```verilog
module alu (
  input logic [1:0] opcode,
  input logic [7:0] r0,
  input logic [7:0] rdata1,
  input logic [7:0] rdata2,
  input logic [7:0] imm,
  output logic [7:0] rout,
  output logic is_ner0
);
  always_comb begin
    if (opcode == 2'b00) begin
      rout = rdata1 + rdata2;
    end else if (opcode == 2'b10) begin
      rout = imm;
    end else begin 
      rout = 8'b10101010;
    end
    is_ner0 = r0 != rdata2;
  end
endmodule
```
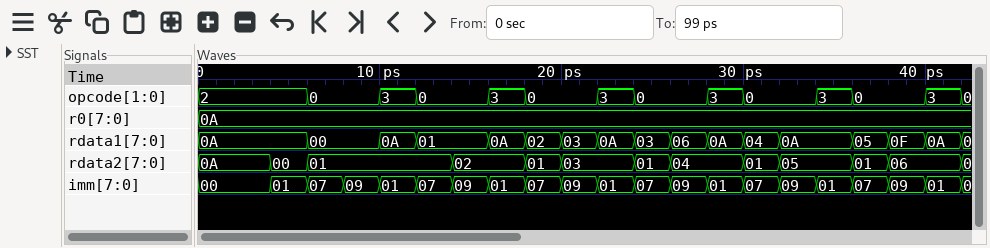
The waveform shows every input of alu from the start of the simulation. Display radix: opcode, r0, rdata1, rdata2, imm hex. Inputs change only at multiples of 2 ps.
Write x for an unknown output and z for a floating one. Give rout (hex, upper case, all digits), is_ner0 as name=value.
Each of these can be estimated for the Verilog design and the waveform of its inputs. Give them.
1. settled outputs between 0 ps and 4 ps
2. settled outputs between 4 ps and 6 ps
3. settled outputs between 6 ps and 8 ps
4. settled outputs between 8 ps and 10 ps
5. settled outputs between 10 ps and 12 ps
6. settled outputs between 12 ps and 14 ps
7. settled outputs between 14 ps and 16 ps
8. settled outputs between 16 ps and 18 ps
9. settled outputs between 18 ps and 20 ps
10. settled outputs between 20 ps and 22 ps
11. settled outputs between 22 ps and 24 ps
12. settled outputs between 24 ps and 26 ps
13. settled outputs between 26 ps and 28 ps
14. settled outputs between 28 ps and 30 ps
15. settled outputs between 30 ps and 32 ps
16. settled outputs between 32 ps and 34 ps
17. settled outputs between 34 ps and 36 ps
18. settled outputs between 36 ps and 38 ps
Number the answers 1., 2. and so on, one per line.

1. rout=00, is_ner0=0
2. rout=01, is_ner0=1
3. rout=01, is_ner0=1
4. rout=01, is_ner0=1
5. rout=AA, is_ner0=1
6. rout=02, is_ner0=1
7. rout=03, is_ner0=1
8. rout=AA, is_ner0=1
9. rout=03, is_ner0=1
10. rout=06, is_ner0=1
11. rout=AA, is_ner0=1
12. rout=04, is_ner0=1
13. rout=0A, is_ner0=1
14. rout=AA, is_ner0=1
15. rout=05, is_ner0=1
16. rout=0F, is_ner0=1
17. rout=AA, is_ner0=1
18. rout=06, is_ner0=1
